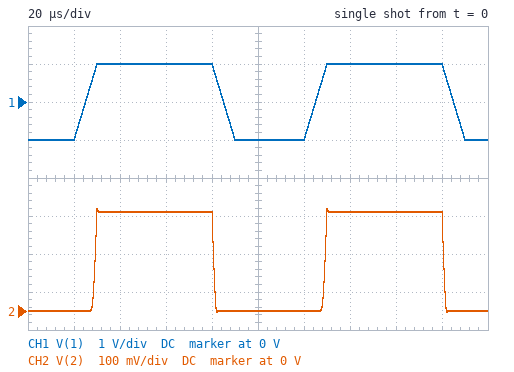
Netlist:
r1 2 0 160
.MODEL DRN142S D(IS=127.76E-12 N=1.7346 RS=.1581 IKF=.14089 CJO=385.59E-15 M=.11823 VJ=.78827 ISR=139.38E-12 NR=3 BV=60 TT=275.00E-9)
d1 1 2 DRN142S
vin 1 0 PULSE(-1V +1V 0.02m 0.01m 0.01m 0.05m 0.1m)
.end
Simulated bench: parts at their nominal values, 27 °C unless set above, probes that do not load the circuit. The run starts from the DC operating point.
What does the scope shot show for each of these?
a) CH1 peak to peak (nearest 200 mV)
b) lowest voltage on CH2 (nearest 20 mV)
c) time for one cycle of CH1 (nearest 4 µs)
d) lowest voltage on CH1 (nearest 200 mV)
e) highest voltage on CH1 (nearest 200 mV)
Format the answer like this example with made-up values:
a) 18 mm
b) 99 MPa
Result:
a) 2.0 V
b) 0 V
c) 100 µs
d) -1.0 V
e) 1.0 V
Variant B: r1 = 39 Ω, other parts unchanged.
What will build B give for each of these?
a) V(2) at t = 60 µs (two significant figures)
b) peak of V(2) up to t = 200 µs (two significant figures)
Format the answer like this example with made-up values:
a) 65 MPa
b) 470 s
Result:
a) 200 mV
b) 210 mV
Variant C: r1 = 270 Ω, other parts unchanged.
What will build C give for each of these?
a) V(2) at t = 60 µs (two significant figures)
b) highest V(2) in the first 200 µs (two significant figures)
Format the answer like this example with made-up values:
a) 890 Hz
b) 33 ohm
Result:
a) 280 mV
b) 290 mV
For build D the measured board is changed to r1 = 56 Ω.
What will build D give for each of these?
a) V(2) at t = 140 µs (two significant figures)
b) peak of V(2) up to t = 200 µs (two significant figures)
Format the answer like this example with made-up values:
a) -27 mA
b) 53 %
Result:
a) 220 mV
b) 230 mV
